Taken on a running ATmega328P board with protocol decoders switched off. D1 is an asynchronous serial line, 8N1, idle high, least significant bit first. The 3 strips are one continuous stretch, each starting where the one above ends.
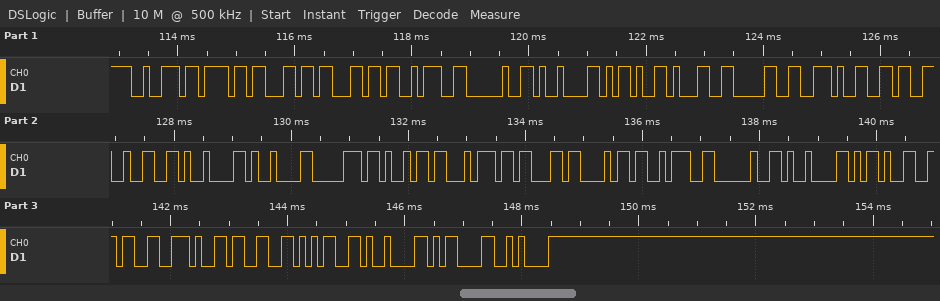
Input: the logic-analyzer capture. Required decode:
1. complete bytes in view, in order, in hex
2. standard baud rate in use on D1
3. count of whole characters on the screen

72 6F 6C 6C 3A 20 09 2D 31 30 2E 36 32 09 09 70 69 74 63 68 3A 20 09 2D 36 2E 33 35 09 0D 0A
9600 baud
31
